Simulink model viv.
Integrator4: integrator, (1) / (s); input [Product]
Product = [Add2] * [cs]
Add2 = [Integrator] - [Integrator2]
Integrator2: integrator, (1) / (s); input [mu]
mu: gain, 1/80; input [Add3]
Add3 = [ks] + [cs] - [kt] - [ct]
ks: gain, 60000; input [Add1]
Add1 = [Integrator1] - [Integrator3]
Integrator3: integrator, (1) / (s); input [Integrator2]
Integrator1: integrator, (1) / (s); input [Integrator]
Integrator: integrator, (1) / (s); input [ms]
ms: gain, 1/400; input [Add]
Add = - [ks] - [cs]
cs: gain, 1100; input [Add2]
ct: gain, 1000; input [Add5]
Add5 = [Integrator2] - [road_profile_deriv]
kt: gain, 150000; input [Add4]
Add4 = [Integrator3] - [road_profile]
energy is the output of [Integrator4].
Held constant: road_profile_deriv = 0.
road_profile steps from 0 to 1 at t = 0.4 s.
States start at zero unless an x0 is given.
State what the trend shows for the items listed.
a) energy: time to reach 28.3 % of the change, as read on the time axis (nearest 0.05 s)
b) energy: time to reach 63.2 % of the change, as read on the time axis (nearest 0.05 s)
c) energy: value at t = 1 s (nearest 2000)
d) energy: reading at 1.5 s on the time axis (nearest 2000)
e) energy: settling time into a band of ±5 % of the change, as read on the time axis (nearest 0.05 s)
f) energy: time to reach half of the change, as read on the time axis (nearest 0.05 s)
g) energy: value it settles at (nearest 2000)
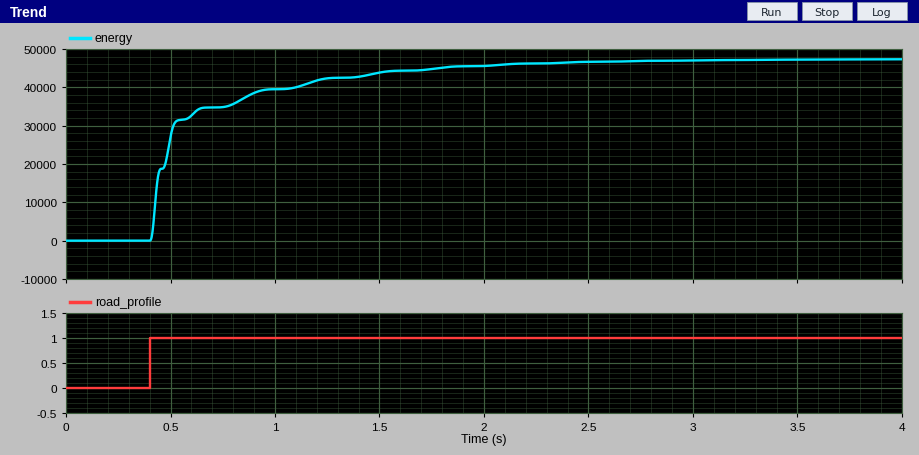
0.45 s
0.50 s
40000
44000
1.80 s
0.50 s
48000
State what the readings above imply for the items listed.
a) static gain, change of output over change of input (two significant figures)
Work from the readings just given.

48000
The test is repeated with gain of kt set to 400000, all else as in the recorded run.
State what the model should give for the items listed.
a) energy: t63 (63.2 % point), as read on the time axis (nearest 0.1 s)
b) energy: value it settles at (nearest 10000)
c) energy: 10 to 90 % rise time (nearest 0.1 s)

0.5 s
120000
0.4 s
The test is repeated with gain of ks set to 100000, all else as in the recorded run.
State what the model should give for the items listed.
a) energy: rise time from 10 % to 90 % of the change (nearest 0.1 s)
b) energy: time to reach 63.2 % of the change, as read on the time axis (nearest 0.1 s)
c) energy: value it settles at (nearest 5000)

1.2 s
0.6 s
45000
